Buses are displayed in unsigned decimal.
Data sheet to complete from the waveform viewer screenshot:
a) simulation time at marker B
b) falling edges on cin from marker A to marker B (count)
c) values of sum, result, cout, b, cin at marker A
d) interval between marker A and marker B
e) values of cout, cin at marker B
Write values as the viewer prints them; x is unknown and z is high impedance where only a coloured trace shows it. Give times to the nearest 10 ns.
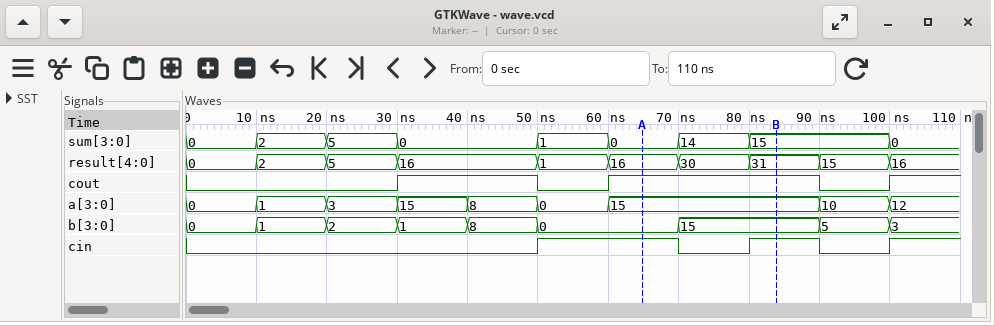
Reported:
80 ns
1
sum=0, result=16, cout=1, b=0, cin=1
20 ns
cout=1, cin=1
